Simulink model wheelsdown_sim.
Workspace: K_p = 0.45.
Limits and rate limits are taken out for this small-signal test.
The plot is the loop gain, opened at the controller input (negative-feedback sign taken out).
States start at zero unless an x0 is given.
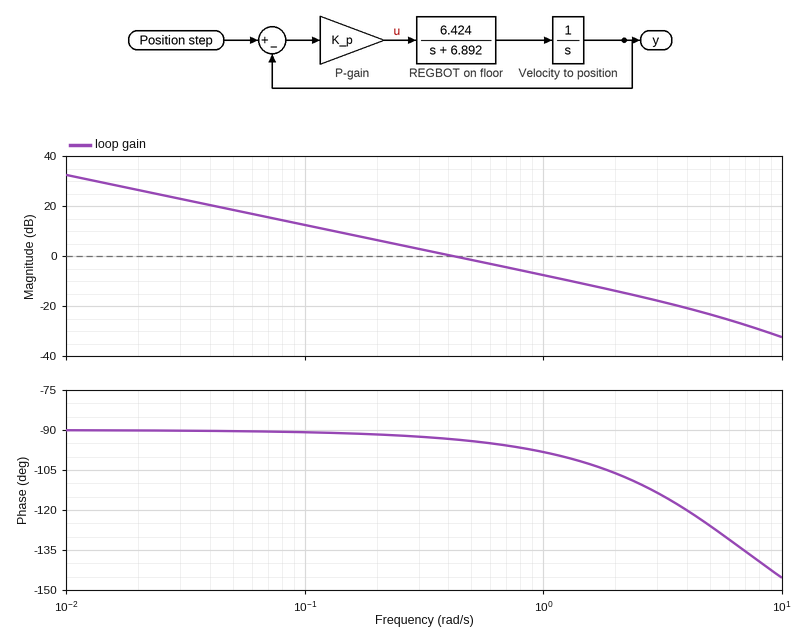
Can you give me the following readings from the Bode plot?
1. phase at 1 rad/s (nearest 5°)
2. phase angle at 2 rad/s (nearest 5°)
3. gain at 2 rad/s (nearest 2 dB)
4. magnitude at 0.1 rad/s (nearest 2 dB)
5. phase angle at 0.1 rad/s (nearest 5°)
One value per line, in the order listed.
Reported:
-100°
-105°
-14 dB
12 dB
-90°
